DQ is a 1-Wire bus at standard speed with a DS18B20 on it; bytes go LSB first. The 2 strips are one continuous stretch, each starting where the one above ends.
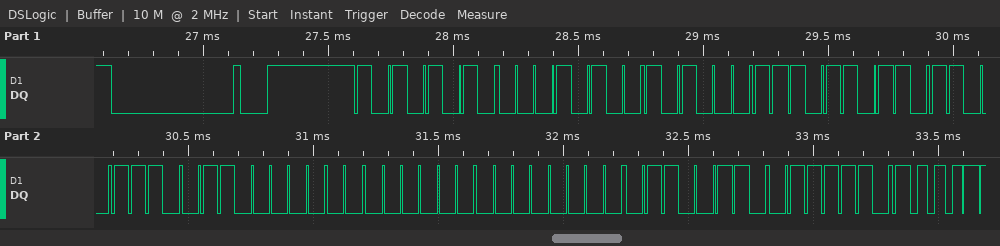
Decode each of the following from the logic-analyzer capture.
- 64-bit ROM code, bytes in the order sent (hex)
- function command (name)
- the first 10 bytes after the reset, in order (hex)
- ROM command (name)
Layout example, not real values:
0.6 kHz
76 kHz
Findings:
28 C5 6D 73 06 00 00 66
Read Scratchpad
55 28 C5 6D 73 06 00 00 66 BE
Match ROM
